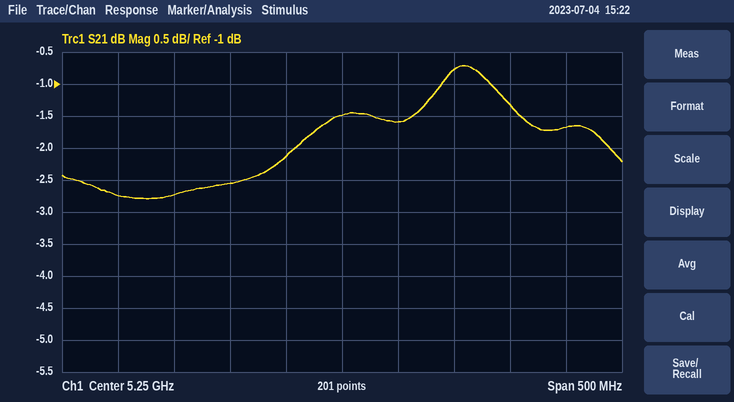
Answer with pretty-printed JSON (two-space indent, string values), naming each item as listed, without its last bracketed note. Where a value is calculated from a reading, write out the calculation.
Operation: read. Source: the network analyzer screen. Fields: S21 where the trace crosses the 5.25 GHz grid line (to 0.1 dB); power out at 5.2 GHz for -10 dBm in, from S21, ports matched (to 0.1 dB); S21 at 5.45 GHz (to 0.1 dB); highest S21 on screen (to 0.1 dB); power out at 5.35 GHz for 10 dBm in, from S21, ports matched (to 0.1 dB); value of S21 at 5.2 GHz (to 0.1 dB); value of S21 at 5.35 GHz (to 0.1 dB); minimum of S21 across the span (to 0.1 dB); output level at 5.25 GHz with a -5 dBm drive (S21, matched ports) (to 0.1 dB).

{
  "S21 where the trace crosses the 5.25 GHz grid line": "-1.5 dB",
  "power out at 5.2 GHz for -10 dBm in, from S21, ports matched": "-10 dBm + (-2.1 dB) = -12.1 dBm",
  "S21 at 5.45 GHz": "-1.7 dB",
  "highest S21 on screen": "-0.7 dB",
  "power out at 5.35 GHz for 10 dBm in, from S21, ports matched": "10 dBm + (-0.8 dB) = 9.2 dBm",
  "value of S21 at 5.2 GHz": "-2.1 dB",
  "value of S21 at 5.35 GHz": "-0.8 dB",
  "minimum of S21 across the span": "-2.8 dB",
  "output level at 5.25 GHz with a -5 dBm drive (S21, matched ports)": "-5 dBm + (-1.5 dB) = -6.5 dBm"
}
